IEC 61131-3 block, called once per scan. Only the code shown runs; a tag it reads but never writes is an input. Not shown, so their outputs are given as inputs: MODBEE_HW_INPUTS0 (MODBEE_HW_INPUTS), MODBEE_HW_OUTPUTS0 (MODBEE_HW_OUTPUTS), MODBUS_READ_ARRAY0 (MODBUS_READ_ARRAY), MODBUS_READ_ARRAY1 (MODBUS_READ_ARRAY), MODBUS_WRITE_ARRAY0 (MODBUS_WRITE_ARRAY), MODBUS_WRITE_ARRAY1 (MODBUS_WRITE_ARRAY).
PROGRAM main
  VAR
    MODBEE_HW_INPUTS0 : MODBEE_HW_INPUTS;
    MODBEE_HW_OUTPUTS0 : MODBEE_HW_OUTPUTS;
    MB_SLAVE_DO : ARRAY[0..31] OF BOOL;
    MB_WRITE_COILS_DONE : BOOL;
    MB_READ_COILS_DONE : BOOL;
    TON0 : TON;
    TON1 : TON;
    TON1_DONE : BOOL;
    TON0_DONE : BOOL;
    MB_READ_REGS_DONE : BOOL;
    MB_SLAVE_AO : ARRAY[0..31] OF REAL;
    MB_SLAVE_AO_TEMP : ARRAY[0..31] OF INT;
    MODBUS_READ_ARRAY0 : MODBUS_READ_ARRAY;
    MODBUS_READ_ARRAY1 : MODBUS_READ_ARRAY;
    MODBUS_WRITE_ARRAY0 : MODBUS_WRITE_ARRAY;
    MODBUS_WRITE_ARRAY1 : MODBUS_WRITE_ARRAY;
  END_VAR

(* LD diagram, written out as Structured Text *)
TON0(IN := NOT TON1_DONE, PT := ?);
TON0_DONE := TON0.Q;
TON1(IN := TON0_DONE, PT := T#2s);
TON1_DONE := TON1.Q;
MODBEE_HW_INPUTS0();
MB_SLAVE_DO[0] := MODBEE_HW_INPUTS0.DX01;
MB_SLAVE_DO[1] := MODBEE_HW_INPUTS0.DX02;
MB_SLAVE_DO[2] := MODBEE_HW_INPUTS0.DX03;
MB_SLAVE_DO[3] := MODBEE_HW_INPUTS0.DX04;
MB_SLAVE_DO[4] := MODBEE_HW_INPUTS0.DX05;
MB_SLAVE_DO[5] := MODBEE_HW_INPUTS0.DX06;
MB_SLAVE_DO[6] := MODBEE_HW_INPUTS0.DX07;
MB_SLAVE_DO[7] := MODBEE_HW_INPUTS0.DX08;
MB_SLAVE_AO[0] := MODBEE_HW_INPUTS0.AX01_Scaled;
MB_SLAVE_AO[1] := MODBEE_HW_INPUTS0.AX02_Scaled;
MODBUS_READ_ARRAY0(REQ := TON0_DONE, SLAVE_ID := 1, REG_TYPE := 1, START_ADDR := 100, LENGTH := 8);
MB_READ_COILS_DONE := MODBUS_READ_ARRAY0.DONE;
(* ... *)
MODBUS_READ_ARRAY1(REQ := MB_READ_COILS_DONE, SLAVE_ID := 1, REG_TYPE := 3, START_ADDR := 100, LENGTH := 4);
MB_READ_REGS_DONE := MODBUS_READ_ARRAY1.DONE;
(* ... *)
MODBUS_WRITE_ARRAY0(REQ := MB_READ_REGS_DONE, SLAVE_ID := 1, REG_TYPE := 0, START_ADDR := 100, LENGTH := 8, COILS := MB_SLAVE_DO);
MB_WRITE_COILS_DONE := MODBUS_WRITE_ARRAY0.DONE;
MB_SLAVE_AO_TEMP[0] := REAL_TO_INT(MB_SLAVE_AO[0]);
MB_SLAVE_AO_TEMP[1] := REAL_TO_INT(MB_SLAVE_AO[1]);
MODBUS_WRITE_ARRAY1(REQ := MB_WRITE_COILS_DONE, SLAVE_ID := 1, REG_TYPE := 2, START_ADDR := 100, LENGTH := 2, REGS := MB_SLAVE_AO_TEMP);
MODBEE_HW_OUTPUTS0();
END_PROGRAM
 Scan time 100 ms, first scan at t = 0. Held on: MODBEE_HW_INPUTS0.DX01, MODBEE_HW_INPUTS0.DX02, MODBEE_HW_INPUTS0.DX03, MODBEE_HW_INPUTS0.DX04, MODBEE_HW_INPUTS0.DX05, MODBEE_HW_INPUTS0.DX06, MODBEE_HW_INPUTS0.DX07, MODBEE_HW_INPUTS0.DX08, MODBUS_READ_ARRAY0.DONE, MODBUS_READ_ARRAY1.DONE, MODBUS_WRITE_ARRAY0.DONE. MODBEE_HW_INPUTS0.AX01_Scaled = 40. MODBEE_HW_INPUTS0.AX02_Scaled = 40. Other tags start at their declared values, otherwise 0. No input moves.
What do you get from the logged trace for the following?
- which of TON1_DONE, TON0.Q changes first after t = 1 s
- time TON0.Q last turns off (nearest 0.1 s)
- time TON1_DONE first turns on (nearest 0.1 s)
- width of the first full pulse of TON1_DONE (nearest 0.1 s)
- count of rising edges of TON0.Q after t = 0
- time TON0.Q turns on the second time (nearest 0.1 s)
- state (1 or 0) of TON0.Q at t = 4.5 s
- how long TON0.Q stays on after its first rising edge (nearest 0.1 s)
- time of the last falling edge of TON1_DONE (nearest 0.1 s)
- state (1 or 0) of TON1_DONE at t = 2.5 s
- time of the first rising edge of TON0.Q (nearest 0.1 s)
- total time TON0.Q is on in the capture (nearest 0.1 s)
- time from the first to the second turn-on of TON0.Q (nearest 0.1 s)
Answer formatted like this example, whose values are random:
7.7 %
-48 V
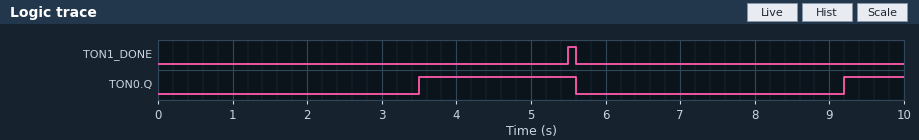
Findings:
TON0.Q
5.6 s
5.5 s
0.1 s
2
9.2 s
1
2.1 s
5.6 s
0
3.5 s
2.9 s
5.7 s
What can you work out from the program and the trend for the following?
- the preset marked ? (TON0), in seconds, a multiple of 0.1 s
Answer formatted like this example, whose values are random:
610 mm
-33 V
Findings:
3.5 s
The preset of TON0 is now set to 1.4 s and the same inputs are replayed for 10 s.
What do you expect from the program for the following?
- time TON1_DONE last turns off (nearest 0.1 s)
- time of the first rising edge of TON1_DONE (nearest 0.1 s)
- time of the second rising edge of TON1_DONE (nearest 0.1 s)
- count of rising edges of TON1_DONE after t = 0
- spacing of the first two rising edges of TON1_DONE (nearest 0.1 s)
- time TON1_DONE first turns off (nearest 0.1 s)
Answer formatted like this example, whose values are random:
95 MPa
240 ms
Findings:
7.1 s
3.4 s
7.0 s
2
3.6 s
3.5 s
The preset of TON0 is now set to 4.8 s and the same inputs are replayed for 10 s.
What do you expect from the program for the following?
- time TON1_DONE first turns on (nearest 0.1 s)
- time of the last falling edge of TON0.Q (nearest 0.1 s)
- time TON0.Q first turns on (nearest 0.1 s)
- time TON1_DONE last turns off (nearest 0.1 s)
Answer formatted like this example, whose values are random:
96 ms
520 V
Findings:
6.8 s
6.9 s
4.8 s
6.9 s
